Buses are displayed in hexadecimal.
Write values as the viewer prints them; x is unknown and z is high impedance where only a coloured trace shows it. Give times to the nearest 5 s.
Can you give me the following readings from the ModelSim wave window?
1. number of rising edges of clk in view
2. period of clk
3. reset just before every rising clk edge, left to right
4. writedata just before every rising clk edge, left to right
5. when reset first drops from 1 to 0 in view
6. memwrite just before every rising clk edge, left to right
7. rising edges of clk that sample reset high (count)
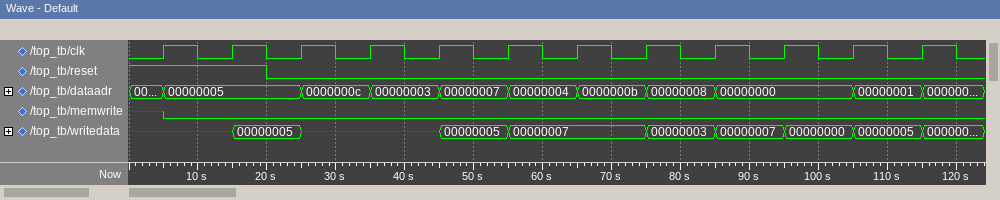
12
10 s
1 1 0 0 0 0 0 0 0 0 0 0
x, x, 00000005, x, x, 00000005, 00000007, 00000007, 00000003, 00000007, 00000000, 00000005
20 s
x 0 0 0 0 0 0 0 0 0 0 0
2
